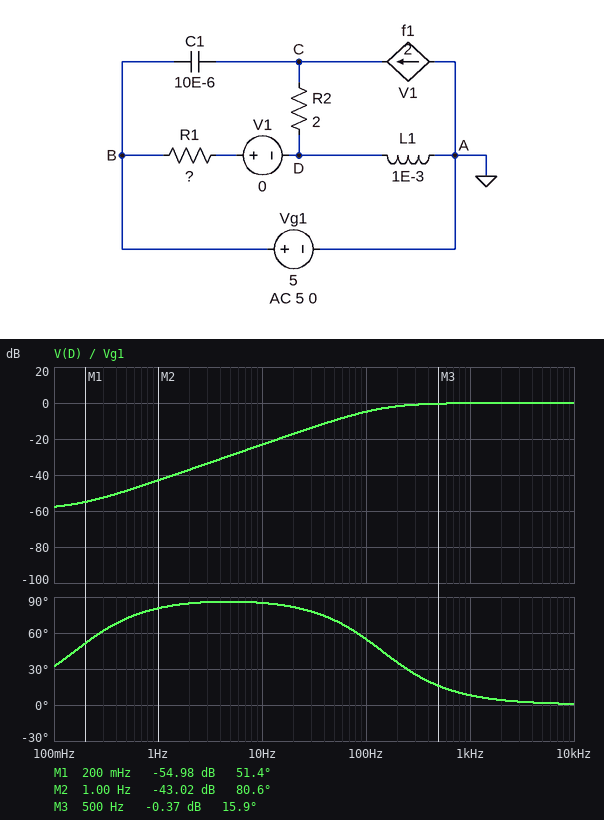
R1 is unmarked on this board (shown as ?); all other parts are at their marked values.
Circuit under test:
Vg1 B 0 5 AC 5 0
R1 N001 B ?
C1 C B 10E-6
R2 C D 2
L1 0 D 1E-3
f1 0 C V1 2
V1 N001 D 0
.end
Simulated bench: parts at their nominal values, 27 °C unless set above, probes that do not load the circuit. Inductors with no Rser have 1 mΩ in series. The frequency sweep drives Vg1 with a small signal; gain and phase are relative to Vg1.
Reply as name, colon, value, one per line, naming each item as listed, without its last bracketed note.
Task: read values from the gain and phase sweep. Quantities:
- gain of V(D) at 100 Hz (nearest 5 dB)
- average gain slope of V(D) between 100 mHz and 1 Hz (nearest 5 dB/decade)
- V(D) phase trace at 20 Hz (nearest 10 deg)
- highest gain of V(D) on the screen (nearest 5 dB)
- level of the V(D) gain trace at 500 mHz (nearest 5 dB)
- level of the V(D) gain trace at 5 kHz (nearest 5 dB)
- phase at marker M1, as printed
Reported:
gain of V(D) at 100 Hz: -5 dB
average gain slope of V(D) between 100 mHz and 1 Hz: 15 dB/decade
V(D) phase trace at 20 Hz: 80 deg
highest gain of V(D) on the screen: 0 dB
level of the V(D) gain trace at 500 mHz: -50 dB
level of the V(D) gain trace at 5 kHz: 0 dB
phase at marker M1, as printed: 51.4 deg
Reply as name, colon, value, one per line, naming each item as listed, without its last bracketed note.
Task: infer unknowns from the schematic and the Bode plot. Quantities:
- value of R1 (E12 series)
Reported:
value of R1: 2.7 Ω
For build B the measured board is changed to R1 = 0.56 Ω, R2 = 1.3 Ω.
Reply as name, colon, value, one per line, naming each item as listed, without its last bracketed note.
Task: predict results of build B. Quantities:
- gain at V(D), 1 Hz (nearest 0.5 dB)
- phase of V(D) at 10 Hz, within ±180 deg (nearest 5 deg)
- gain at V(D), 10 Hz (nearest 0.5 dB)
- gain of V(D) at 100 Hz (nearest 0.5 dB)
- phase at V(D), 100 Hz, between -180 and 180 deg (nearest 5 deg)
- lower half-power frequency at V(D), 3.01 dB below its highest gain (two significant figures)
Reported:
gain at V(D), 1 Hz: -29.5 dB
phase of V(D) at 10 Hz, within ±180 deg: 70 deg
gain at V(D), 10 Hz: -10.0 dB
gain of V(D) at 100 Hz: -0.5 dB
phase at V(D), 100 Hz, between -180 and 180 deg: 15 deg
lower half-power frequency at V(D), 3.01 dB below its highest gain: 30 Hz
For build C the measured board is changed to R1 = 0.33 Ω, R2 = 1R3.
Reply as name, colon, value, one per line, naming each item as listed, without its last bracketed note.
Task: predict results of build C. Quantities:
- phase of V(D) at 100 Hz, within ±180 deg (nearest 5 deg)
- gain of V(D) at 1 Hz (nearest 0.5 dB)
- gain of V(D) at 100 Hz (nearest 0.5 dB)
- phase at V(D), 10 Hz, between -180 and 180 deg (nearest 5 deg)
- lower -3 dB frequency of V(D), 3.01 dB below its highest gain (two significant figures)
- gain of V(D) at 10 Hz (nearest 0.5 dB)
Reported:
phase of V(D) at 100 Hz, within ±180 deg: 10 deg
gain of V(D) at 1 Hz: -25.0 dB
gain of V(D) at 100 Hz: 0 dB
phase at V(D), 10 Hz, between -180 and 180 deg: 60 deg
lower -3 dB frequency of V(D), 3.01 dB below its highest gain: 18 Hz
gain of V(D) at 10 Hz: -6.0 dB
